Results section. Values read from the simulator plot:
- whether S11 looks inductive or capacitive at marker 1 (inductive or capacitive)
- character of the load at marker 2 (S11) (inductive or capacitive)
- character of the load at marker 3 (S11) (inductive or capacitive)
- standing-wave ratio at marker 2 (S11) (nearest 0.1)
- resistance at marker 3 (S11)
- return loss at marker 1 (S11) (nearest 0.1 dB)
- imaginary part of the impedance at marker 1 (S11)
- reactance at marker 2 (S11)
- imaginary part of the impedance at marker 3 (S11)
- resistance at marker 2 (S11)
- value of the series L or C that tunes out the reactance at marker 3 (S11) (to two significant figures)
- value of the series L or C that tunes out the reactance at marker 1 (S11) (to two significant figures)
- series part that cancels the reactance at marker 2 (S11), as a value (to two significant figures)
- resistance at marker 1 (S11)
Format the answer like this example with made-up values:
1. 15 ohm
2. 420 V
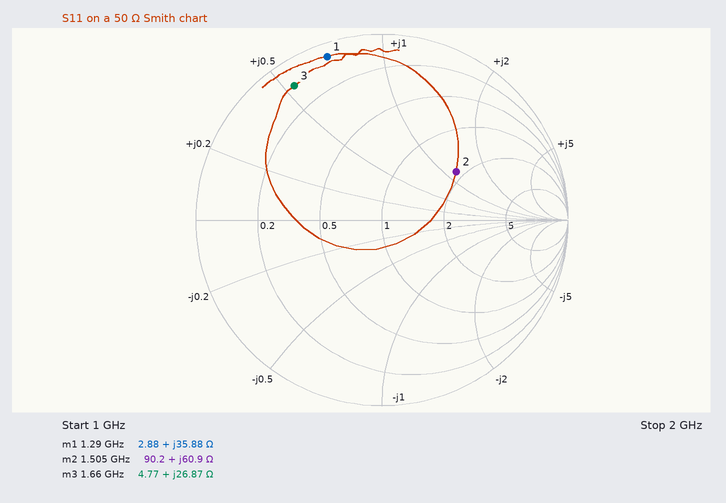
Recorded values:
1. inductive
2. inductive
3. inductive
4. 2.8
5. 4.77 Ω
6. 0.7 dB
7. +35.88 Ω
8. +60.9 Ω
9. +26.87 Ω
10. 90.2 Ω
11. 3.6 pF
12. 3.4 pF
13. 1.7 pF
14. 2.88 Ω
